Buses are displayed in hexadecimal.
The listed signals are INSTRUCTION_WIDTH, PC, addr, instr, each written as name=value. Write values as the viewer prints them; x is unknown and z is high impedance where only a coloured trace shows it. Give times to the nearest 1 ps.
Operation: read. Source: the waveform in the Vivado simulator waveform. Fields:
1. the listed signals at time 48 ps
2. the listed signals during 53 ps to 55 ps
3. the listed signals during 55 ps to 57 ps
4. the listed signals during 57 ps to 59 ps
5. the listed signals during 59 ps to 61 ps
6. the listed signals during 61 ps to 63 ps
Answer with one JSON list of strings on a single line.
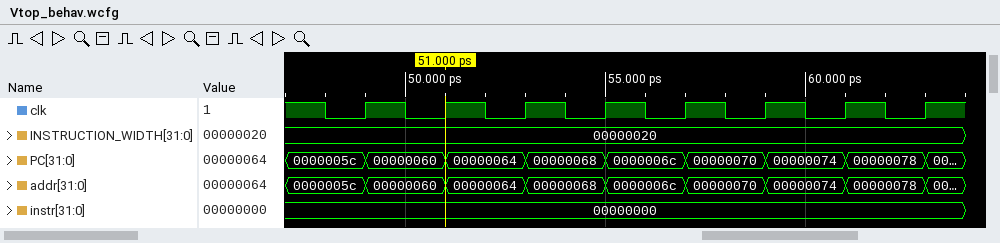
["INSTRUCTION_WIDTH=00000020, PC=0000005c, addr=0000005c, instr=00000000", "INSTRUCTION_WIDTH=00000020, PC=00000068, addr=00000068, instr=00000000", "INSTRUCTION_WIDTH=00000020, PC=0000006c, addr=0000006c, instr=00000000", "INSTRUCTION_WIDTH=00000020, PC=00000070, addr=00000070, instr=00000000", "INSTRUCTION_WIDTH=00000020, PC=00000074, addr=00000074, instr=00000000", "INSTRUCTION_WIDTH=00000020, PC=00000078, addr=00000078, instr=00000000"]
